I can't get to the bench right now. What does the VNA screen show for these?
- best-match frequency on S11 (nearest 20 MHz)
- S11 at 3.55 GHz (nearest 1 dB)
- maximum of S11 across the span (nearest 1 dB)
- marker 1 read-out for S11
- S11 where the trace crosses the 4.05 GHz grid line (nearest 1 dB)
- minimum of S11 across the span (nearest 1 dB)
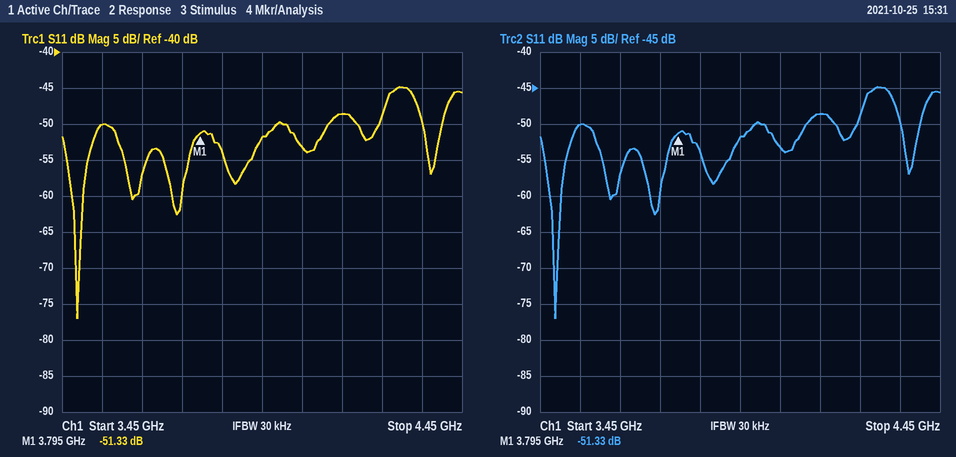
3.48 GHz
-50 dB
-45 dB
-51.33 dB
-53 dB
-77 dB
